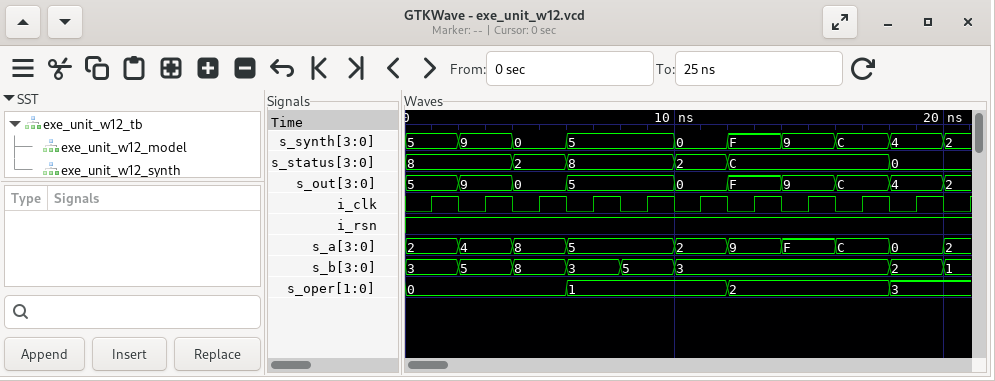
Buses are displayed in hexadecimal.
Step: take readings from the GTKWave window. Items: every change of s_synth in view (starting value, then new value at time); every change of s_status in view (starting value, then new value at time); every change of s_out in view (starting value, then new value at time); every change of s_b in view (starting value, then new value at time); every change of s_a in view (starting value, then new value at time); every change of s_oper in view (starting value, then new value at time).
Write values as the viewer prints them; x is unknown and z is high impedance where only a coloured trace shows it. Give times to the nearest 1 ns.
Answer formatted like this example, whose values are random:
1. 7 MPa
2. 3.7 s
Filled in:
1. 5, 9 at 2 ns, 0 at 4 ns, 5 at 6 ns, 0 at 10 ns, F at 12 ns, 9 at 14 ns, C at 16 ns, 4 at 18 ns, 2 at 20 ns
2. 8, 2 at 4 ns, 8 at 6 ns, 2 at 10 ns, C at 12 ns, 0 at 18 ns
3. 5, 9 at 2 ns, 0 at 4 ns, 5 at 6 ns, 0 at 10 ns, F at 12 ns, 9 at 14 ns, C at 16 ns, 4 at 18 ns, 2 at 20 ns
4. 3, 5 at 2 ns, 8 at 4 ns, 3 at 6 ns, 5 at 8 ns, 3 at 10 ns, 2 at 18 ns, 1 at 20 ns
5. 2, 4 at 2 ns, 8 at 4 ns, 5 at 6 ns, 2 at 10 ns, 9 at 12 ns, F at 14 ns, C at 16 ns, 0 at 18 ns, 2 at 20 ns
6. 0, 1 at 6 ns, 2 at 12 ns, 3 at 18 ns
